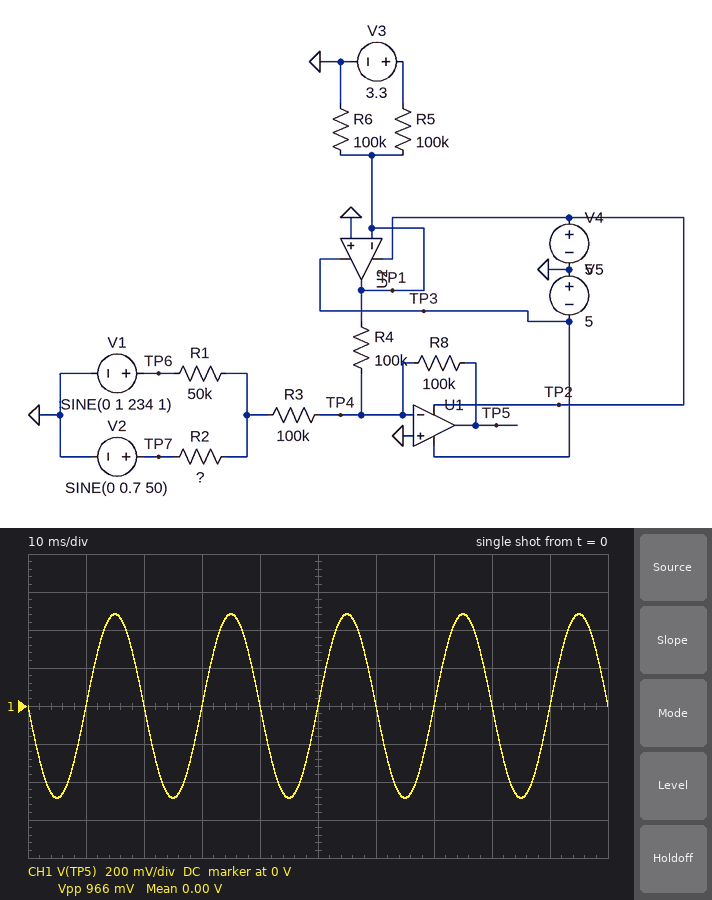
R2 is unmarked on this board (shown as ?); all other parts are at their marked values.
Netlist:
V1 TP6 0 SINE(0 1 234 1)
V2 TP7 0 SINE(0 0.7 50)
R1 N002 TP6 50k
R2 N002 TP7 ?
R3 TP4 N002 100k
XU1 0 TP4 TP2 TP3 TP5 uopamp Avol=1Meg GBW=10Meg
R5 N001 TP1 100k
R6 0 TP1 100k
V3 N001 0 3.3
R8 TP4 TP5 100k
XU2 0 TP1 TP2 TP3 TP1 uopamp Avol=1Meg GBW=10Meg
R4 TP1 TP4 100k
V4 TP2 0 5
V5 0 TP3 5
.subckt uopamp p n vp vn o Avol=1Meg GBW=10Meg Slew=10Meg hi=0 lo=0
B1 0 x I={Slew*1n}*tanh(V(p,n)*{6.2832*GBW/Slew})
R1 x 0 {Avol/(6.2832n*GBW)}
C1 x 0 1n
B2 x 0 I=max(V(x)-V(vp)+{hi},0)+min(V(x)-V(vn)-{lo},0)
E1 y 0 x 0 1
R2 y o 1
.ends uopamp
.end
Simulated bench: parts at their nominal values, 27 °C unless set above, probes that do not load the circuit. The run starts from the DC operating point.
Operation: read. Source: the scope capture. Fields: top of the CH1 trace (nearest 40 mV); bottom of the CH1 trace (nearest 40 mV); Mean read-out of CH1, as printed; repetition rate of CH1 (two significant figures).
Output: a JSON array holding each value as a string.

["480 mV", "-480 mV", "0.00 V", "50 Hz"]
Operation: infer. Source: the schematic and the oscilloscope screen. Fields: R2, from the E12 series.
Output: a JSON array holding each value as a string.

["15 kΩ"]
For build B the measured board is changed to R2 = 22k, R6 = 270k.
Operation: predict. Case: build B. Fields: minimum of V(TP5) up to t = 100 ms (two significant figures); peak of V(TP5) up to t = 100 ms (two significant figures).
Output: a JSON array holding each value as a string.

["-420 mV", "420 mV"]
